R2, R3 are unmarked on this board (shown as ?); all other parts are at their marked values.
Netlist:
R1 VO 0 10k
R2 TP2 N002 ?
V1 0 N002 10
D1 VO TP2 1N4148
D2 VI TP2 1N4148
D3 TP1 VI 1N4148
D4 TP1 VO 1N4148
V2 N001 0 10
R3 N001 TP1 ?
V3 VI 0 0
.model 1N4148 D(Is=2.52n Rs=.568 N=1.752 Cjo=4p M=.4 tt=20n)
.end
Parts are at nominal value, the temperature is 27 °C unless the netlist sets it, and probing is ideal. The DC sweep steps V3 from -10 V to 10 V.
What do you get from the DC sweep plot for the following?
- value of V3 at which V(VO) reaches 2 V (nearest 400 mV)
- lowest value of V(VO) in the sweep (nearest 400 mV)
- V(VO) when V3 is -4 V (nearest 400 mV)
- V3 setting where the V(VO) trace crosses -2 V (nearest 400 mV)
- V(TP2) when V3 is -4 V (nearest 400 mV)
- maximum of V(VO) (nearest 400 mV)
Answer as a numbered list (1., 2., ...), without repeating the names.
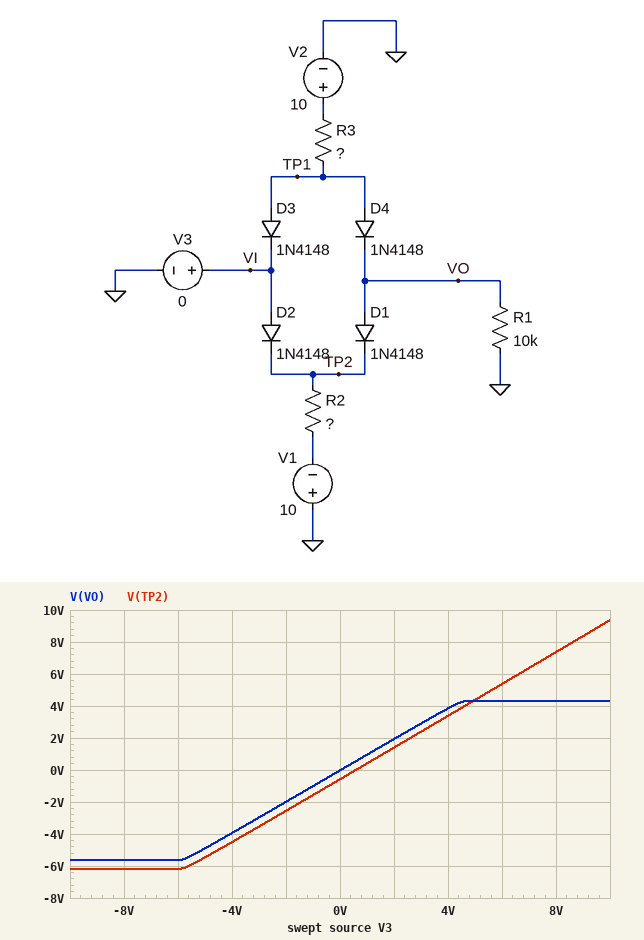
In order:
1. 2.0 V
2. -5.6 V
3. -4.0 V
4. -2.0 V
5. -4.4 V
6. 4.4 V
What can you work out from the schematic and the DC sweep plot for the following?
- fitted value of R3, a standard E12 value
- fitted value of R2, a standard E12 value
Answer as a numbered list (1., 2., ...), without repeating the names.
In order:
1. 12 kΩ
2. 6.8 kΩ
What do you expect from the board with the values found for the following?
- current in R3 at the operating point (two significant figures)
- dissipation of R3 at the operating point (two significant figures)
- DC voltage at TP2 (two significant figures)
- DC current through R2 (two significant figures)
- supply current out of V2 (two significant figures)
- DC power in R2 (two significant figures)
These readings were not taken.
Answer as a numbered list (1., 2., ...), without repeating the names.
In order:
1. 790 µA
2. 7.5 mW
3. -580 mV
4. 1.4 mA
5. 790 µA
6. 13 mW
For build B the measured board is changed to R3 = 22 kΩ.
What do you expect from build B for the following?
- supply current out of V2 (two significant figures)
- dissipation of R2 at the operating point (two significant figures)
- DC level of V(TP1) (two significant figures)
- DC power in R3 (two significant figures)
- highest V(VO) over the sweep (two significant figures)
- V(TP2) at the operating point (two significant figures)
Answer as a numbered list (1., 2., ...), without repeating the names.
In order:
1. 430 µA
2. 13 mW
3. 480 mV
4. 4.1 mW
5. 3.0 V
6. -590 mV
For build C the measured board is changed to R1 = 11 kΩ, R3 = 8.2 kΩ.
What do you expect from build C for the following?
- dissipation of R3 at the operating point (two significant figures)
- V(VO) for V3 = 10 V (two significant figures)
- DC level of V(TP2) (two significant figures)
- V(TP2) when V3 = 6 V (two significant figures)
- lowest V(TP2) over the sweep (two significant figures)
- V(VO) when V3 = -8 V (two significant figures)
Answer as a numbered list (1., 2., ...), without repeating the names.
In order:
1. 11 mW
2. 5.4 V
3. -570 mV
4. 5.4 V
5. -6.4 V
6. -5.8 V
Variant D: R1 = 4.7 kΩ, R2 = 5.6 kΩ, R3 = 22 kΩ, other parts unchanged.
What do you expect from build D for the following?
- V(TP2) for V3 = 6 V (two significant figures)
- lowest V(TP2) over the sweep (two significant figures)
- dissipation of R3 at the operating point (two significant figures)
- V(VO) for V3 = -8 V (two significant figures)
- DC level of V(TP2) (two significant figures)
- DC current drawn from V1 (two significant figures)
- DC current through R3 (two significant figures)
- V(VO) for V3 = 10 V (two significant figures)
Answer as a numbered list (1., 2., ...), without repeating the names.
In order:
1. 5.4 V
2. -4.9 V
3. 4.1 mW
4. -4.3 V
5. -600 mV
6. 1.7 mA
7. 430 µA
8. 1.7 V
